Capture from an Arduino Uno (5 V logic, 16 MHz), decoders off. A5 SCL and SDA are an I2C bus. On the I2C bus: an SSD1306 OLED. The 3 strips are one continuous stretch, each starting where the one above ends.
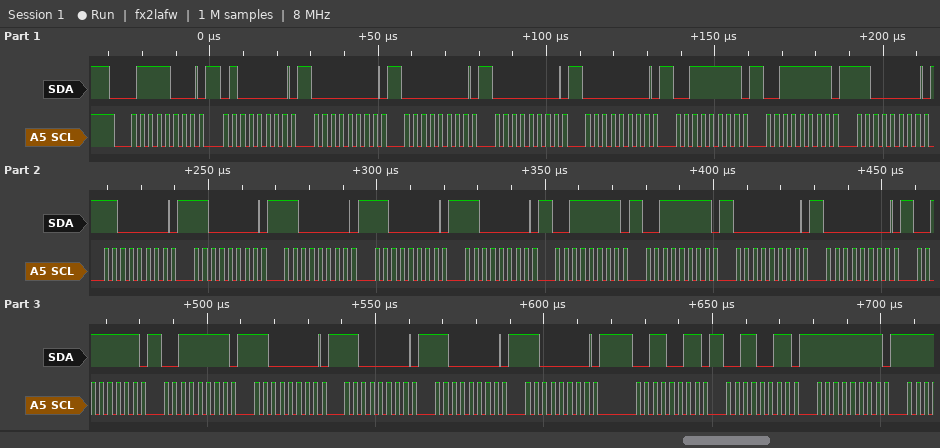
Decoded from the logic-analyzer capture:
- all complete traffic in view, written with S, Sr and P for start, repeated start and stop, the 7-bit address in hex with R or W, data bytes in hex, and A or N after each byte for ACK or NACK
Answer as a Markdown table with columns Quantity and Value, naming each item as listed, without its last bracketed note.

| Quantity | Value |
|---|---|
| all complete traffic in view, written with S, Sr and P for start, repeated start and stop, the 7-bit address in hex with R or W, data bytes in hex, and A or N after each byte for ACK or NACK | S 3CW A 40 A 00 A 00 A 00 A 00 A 3F A 3F A C0 A C0 A C0 A C0 A C0 A C0 A 3F A 3F A 00 A 00 A 3F A 3F A C0 A C0 A C0 A C0 A 33 A 33 A FF A |
